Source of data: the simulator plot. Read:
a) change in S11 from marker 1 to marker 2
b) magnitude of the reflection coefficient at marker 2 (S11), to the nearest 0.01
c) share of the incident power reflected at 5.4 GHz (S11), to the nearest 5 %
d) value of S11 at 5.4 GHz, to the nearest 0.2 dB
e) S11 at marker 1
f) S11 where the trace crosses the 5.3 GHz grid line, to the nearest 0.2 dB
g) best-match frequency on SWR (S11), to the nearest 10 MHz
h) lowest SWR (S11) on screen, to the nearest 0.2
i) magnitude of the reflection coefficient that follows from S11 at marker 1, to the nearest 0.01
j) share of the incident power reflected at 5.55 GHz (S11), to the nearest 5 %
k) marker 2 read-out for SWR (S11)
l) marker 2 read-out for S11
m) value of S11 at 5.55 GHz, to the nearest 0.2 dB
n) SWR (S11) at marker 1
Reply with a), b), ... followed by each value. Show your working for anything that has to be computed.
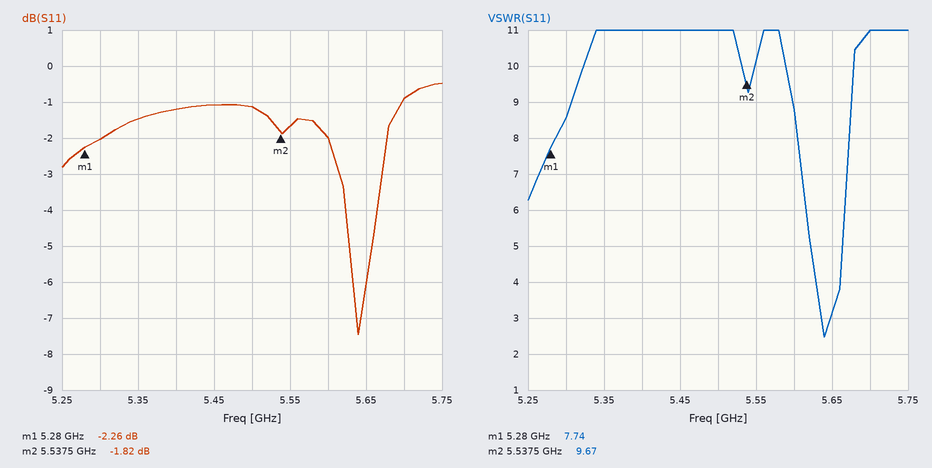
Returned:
a) -1.82 − (-2.26) = 0.44 dB
b) 10^(-1.82/20) ≈ 0.81
c) 10^(-1.2/10) ≈ 75.9 %, so 75 % to the nearest 5 %
d) -1.2 dB
e) -2.26 dB
f) -2.0 dB
g) 5.64 GHz
h) 2.4
i) 10^(-2.26/20) ≈ 0.77
j) 10^(-1.6/10) ≈ 69.2 %, so 70 % to the nearest 5 %
k) 9.67
l) -1.82 dB
m) -1.6 dB
n) 7.74
